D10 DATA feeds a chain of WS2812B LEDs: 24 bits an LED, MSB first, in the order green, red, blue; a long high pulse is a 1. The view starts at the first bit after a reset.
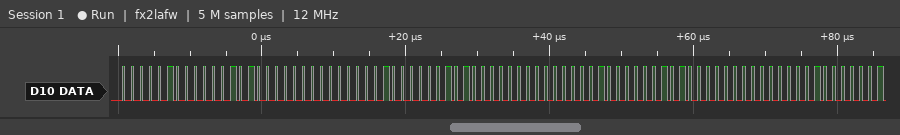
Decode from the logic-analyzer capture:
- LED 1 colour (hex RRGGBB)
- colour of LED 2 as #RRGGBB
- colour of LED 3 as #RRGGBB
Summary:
#0A0400
#0A0400
#0A0400
